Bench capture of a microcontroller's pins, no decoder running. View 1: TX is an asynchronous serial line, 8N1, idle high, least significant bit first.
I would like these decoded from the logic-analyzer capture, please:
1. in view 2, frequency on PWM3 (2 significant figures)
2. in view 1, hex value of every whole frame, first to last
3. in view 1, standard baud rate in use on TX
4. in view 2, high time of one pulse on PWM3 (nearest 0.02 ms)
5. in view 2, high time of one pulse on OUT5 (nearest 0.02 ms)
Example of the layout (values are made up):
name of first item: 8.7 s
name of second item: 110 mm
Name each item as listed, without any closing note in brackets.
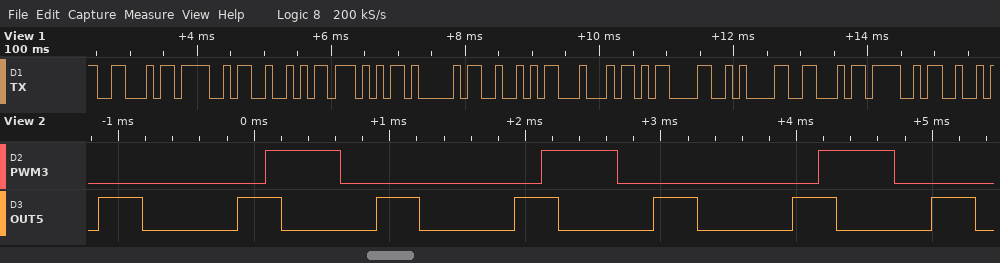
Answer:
in view 2, frequency on PWM3: 490 Hz
in view 1, hex value of every whole frame, first to last: 0x46 0x4F 0x52 0x57 0x41 0x52 0x44 0x0D 0x0A 0x46 0x4F
in view 1, standard baud rate in use on TX: 9600 baud
in view 2, high time of one pulse on PWM3: 0.56 ms
in view 2, high time of one pulse on OUT5: 0.32 ms
